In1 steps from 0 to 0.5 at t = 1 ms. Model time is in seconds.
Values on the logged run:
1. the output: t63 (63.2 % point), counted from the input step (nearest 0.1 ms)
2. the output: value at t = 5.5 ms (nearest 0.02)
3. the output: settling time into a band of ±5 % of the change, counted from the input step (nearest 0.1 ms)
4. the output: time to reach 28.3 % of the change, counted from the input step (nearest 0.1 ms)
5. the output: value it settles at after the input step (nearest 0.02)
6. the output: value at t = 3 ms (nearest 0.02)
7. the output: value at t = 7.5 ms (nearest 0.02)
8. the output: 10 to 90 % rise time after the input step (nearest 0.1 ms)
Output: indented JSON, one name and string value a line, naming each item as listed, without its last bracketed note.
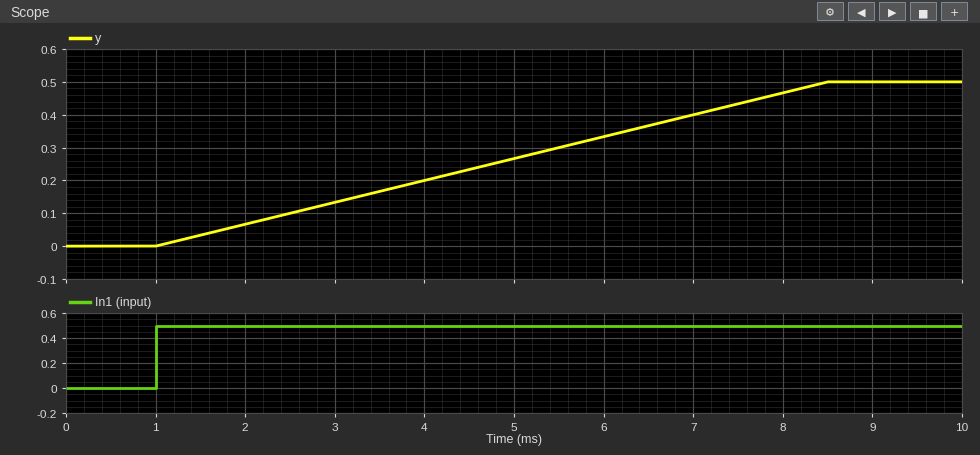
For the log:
{
  "the output: t63 (63.2 % point), counted from the input step": "4.7 ms",
  "the output: value at t = 5.5 ms": "0.30",
  "the output: settling time into a band of ±5 % of the change, counted from the input step": "7.1 ms",
  "the output: time to reach 28.3 % of the change, counted from the input step": "2.1 ms",
  "the output: value it settles at after the input step": "0.50",
  "the output: value at t = 3 ms": "0.14",
  "the output: value at t = 7.5 ms": "0.44",
  "the output: 10 to 90 % rise time after the input step": "6.0 ms"
}
